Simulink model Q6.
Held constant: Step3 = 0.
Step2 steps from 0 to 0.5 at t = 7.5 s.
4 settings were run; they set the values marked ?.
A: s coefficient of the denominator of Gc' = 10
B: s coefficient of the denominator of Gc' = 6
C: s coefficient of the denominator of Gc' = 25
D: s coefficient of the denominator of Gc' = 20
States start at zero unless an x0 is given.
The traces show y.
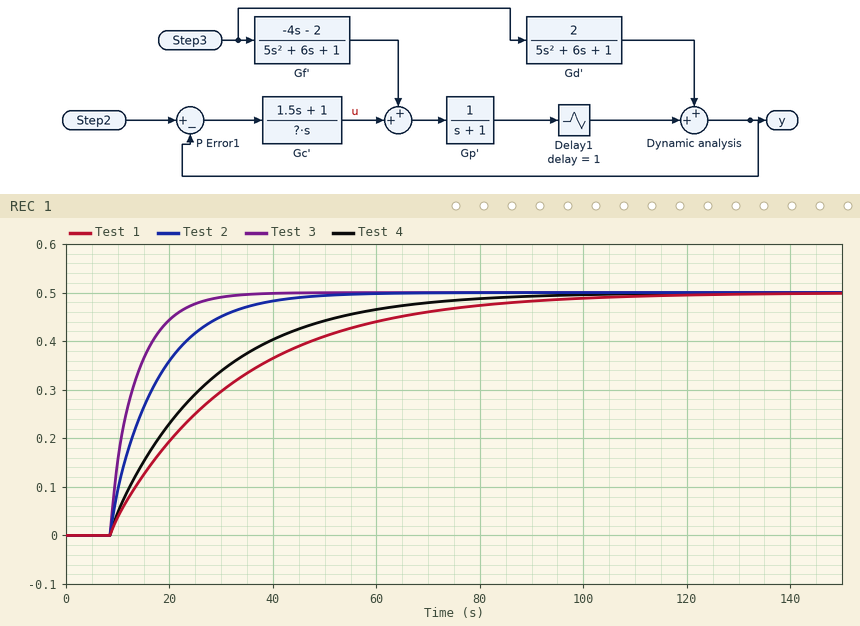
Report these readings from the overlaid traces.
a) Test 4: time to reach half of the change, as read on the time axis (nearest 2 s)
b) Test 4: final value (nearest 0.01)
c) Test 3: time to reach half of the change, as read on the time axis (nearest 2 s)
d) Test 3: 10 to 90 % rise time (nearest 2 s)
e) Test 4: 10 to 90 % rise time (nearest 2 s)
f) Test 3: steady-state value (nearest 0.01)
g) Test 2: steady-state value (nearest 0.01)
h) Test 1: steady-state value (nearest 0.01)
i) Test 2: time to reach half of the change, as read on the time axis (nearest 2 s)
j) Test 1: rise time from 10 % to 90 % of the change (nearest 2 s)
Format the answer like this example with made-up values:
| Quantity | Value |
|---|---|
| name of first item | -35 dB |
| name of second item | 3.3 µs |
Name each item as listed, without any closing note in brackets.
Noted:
| Quantity | Value |
|---|---|
| Test 4: time to reach half of the change, as read on the time axis | 22 s |
| Test 4: final value | 0.50 |
| Test 3: time to reach half of the change, as read on the time axis | 12 s |
| Test 3: 10 to 90 % rise time | 12 s |
| Test 4: 10 to 90 % rise time | 42 s |
| Test 3: steady-state value | 0.50 |
| Test 2: steady-state value | 0.50 |
| Test 1: steady-state value | 0.50 |
| Test 2: time to reach half of the change, as read on the time axis | 14 s |
| Test 1: rise time from 10 % to 90 % of the change | 54 s |
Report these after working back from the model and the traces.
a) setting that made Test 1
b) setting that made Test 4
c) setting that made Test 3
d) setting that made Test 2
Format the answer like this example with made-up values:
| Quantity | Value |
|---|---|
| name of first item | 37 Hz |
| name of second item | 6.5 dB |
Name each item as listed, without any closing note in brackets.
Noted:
| Quantity | Value |
|---|---|
| setting that made Test 1 | C |
| setting that made Test 4 | D |
| setting that made Test 3 | B |
| setting that made Test 2 | A |
